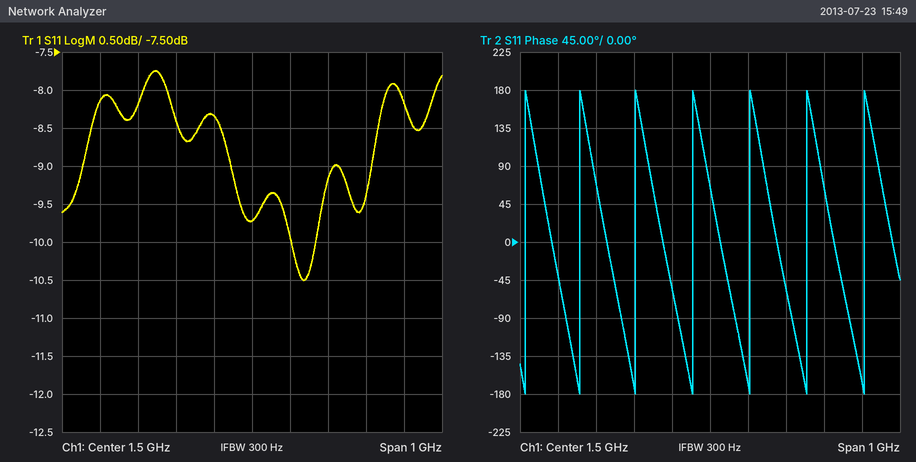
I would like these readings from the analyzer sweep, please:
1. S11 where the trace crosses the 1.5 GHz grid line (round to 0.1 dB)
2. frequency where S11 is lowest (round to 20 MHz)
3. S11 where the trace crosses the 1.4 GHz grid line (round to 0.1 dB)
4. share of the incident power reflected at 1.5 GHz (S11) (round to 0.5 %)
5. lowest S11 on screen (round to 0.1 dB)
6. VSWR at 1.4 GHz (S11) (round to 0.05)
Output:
-9.7 dB
1.64 GHz
-8.3 dB
10.5 %
-10.5 dB
2.25
